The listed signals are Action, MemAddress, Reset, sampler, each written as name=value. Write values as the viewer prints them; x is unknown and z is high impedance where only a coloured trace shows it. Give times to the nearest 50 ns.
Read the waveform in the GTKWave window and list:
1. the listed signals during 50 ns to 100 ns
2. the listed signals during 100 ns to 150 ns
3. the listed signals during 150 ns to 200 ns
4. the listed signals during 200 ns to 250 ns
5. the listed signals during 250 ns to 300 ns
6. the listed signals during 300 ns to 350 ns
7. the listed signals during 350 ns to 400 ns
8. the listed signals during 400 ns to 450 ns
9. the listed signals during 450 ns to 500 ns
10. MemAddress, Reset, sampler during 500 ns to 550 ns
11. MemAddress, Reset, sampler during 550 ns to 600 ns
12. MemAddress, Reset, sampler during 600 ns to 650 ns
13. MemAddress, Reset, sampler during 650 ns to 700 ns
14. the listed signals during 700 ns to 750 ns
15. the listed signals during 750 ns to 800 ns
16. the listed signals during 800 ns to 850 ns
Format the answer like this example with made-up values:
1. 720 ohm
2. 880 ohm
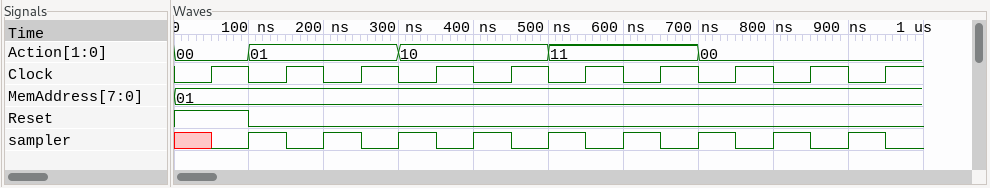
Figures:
1. Action=00, MemAddress=01, Reset=1, sampler=0
2. Action=01, MemAddress=01, Reset=0, sampler=1
3. Action=01, MemAddress=01, Reset=0, sampler=0
4. Action=01, MemAddress=01, Reset=0, sampler=1
5. Action=01, MemAddress=01, Reset=0, sampler=0
6. Action=10, MemAddress=01, Reset=0, sampler=1
7. Action=10, MemAddress=01, Reset=0, sampler=0
8. Action=10, MemAddress=01, Reset=0, sampler=1
9. Action=10, MemAddress=01, Reset=0, sampler=0
10. MemAddress=01, Reset=0, sampler=1
11. MemAddress=01, Reset=0, sampler=0
12. MemAddress=01, Reset=0, sampler=1
13. MemAddress=01, Reset=0, sampler=0
14. Action=00, MemAddress=01, Reset=0, sampler=1
15. Action=00, MemAddress=01, Reset=0, sampler=0
16. Action=00, MemAddress=01, Reset=0, sampler=1
